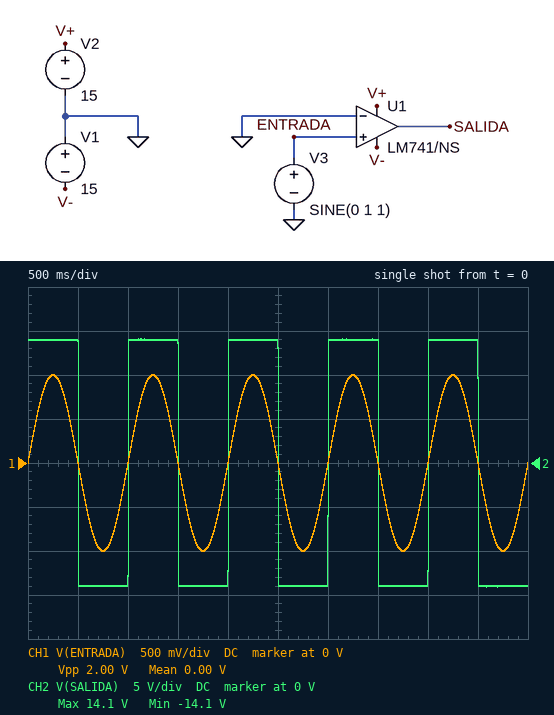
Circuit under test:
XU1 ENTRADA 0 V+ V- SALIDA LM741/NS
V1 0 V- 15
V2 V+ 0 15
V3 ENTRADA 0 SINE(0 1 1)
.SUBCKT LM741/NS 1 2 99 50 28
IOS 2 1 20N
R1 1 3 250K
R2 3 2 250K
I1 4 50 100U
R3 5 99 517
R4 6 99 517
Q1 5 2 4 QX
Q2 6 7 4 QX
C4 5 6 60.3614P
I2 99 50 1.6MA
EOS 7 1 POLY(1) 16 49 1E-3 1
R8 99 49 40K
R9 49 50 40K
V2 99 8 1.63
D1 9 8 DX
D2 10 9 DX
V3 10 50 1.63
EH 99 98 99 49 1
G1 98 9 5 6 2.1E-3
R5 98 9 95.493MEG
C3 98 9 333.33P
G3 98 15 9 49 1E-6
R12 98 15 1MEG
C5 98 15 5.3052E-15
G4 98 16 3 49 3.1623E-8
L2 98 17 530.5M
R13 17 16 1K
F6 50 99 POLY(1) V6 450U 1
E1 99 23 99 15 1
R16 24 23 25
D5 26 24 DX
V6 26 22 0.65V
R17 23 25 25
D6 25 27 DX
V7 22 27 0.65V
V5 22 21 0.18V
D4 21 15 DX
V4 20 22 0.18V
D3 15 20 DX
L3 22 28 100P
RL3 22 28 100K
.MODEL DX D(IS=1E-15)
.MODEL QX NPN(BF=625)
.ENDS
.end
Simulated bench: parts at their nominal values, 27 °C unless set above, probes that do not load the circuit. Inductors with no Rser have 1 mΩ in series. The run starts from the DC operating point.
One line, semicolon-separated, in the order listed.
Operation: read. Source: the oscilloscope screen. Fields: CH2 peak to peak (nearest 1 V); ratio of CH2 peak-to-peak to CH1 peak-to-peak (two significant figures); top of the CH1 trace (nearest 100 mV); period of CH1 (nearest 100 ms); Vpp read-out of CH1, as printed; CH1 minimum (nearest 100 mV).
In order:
28 V; 14; 1.0 V; 1.0 s; 2.00 V; -1.0 V
